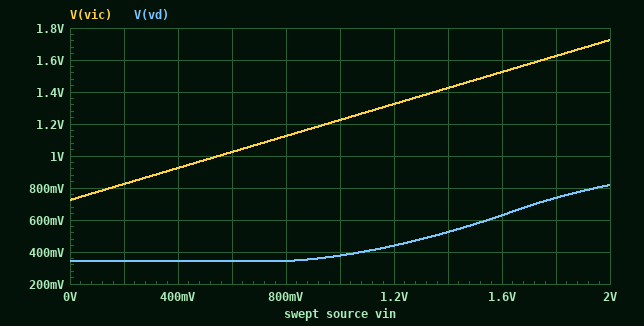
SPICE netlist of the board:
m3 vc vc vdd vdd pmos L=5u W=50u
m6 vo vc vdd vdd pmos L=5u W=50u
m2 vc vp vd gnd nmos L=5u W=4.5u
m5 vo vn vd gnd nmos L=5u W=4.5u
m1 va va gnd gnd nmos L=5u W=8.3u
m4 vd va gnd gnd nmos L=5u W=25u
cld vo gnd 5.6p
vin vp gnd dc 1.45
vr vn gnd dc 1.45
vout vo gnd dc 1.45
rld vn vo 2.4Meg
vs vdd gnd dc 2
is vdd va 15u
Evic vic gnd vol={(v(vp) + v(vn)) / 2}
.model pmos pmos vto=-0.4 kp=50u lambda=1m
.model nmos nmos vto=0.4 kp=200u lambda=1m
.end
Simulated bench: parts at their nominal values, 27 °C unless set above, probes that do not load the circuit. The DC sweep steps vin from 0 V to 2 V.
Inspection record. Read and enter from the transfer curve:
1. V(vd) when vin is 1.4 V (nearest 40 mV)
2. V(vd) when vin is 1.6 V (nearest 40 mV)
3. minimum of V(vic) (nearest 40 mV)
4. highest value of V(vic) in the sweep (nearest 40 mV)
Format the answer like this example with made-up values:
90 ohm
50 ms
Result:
520 mV
640 mV
720 mV
1.72 V
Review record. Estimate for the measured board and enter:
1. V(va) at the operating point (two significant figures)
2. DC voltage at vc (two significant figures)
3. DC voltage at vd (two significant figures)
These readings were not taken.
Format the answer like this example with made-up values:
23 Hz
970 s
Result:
700 mV
1.3 V
550 mV
